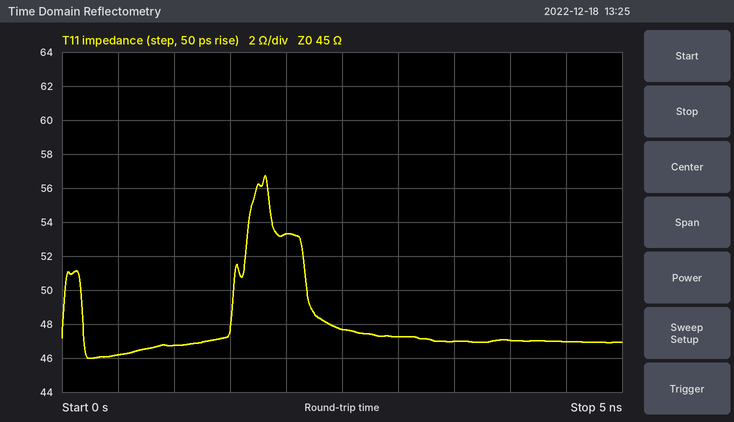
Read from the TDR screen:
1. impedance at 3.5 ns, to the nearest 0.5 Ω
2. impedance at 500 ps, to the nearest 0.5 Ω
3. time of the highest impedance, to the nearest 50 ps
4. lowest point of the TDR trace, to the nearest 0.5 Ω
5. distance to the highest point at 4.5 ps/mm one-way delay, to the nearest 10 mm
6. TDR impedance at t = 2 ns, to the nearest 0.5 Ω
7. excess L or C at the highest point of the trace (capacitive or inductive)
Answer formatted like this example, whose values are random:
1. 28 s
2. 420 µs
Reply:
1. 47.0 Ω
2. 46.0 Ω
3. 1.80 ns
4. 46.0 Ω
5. 200 mm
6. 53.5 Ω
7. inductive
